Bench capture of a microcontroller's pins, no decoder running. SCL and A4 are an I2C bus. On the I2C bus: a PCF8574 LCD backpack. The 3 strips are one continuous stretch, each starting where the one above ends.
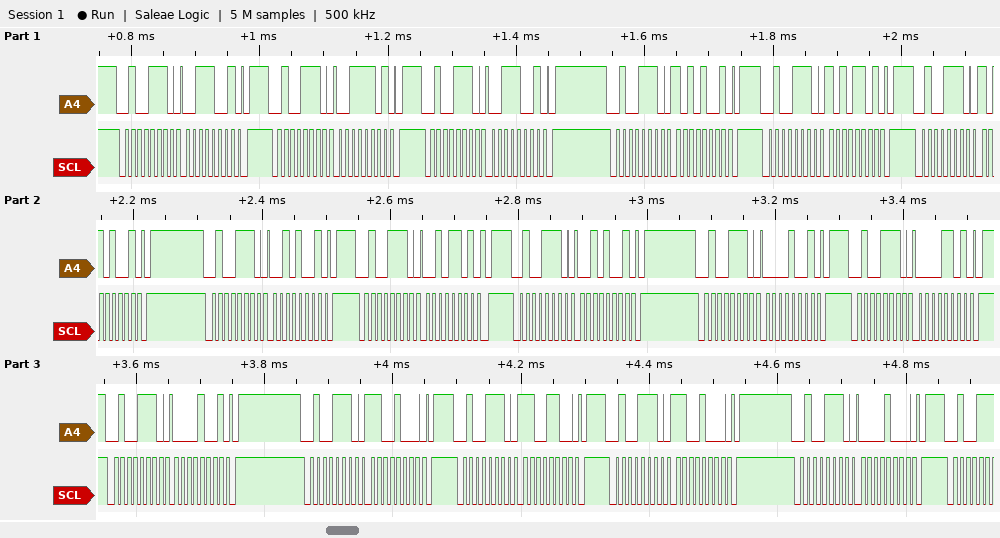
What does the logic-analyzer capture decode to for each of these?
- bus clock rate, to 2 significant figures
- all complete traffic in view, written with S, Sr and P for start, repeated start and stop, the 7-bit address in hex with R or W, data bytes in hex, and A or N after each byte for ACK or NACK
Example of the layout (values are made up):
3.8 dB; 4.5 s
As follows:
100 kHz; S 27W A 39 A P S 27W A 3D A P S 27W A 39 A P S 27W A A9 A P S 27W A AD A P S 27W A A9 A P S 27W A 29 A P S 27W A 2D A P S 27W A 29 A P S 27W A 09 A P S 27W A 0D A P S 27W A 09 A P S 27W A C8 A P S 27W A CC A P S 27W A C8 A P S 27W A 08 A P
